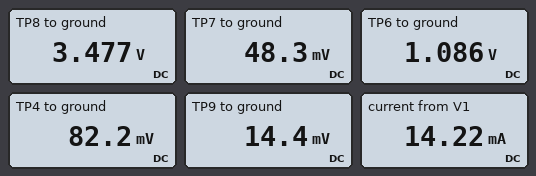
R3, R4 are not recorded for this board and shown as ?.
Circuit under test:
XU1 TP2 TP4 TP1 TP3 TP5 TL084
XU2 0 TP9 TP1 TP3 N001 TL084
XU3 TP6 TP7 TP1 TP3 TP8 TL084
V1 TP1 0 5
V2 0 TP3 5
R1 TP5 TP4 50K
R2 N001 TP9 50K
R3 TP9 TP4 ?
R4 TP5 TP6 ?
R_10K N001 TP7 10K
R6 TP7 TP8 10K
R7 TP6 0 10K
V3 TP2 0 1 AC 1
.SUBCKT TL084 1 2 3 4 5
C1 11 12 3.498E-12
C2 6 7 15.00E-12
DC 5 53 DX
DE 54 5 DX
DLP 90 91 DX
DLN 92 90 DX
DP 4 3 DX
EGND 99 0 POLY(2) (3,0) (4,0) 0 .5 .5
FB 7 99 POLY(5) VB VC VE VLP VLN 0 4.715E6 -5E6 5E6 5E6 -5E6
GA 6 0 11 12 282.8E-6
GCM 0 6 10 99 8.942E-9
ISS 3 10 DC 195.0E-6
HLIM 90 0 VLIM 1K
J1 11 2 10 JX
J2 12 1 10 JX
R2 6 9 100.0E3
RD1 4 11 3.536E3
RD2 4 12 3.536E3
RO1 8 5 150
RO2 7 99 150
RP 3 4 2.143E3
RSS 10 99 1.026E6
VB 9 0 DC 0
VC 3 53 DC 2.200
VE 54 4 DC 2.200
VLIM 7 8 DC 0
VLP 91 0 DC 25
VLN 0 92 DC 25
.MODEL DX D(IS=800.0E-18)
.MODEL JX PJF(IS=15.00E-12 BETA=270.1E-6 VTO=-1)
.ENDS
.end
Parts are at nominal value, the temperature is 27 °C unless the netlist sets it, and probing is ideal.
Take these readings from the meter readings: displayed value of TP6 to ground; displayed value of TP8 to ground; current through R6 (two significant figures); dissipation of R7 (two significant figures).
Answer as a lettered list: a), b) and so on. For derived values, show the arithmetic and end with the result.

a) 1.086 V
b) 3.477 V
c) (3.477 V - 48.3 mV) / 10 kΩ = 340 µA
d) (1.086 V)^2 / 10 kΩ = 120 µW
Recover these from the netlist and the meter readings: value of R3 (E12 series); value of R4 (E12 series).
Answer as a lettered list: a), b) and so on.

a) 1 kΩ
b) 22 kΩ
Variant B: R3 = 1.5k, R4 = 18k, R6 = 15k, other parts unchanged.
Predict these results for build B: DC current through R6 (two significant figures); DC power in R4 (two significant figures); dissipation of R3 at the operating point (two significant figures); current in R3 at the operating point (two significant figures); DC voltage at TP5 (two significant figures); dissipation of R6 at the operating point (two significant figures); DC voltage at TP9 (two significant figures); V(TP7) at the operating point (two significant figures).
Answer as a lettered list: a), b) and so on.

a) 270 µA
b) 280 µW
c) 6.8 µW
d) 67 µA
e) 3.5 V
f) 1.1 mW
g) 7.0 mV
h) -630 mV
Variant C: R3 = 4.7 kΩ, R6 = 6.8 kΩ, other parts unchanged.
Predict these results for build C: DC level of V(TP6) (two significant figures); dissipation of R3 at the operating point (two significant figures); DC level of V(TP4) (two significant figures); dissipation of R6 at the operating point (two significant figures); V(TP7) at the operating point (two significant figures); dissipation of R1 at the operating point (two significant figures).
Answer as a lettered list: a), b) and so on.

a) 1.1 V
b) 19 µW
c) 300 mV
d) 1.1 mW
e) 770 mV
f) 200 µW
